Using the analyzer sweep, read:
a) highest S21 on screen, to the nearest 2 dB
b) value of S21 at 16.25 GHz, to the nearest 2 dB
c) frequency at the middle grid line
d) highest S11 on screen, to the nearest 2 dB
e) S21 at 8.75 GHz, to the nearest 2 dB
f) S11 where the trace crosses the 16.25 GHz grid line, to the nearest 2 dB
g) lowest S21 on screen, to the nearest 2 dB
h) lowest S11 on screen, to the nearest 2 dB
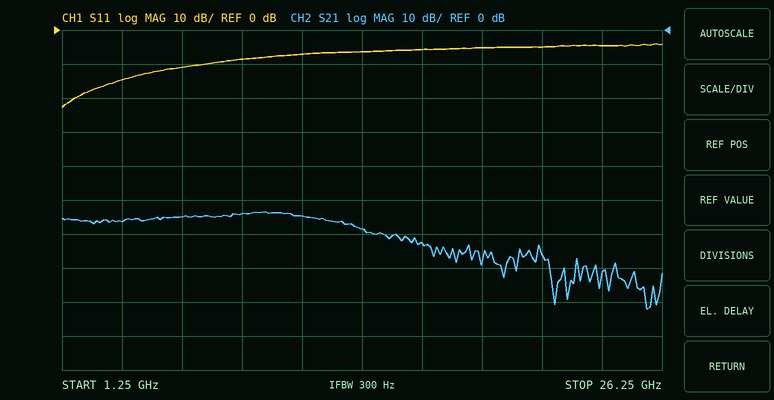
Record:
-54 dB
-62 dB
13.75 GHz
-4 dB
-54 dB
-6 dB
-82 dB
-22 dB
